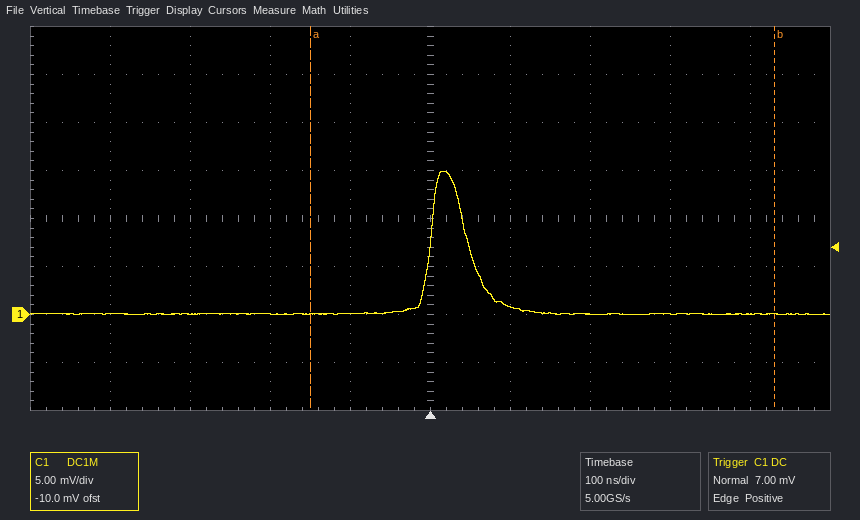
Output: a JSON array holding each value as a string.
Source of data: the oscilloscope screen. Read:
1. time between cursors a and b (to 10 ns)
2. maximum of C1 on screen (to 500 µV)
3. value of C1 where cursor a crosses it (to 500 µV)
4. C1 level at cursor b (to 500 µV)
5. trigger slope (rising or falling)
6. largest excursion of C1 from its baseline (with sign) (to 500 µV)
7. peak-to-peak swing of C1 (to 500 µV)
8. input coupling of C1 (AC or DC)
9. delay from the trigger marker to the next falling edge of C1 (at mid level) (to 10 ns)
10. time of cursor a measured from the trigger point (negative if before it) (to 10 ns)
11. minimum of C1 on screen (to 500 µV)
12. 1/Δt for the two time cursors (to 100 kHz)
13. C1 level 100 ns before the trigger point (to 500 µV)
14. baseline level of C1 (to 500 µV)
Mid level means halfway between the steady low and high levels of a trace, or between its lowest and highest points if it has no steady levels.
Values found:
["580 ns", "15.0 mV", "0.0 mV", "0.0 mV", "rising", "+15.0 mV", "15.0 mV", "DC", "50 ns", "-150 ns", "0.0 mV", "1.7 MHz", "0.0 mV", "0.0 mV"]
